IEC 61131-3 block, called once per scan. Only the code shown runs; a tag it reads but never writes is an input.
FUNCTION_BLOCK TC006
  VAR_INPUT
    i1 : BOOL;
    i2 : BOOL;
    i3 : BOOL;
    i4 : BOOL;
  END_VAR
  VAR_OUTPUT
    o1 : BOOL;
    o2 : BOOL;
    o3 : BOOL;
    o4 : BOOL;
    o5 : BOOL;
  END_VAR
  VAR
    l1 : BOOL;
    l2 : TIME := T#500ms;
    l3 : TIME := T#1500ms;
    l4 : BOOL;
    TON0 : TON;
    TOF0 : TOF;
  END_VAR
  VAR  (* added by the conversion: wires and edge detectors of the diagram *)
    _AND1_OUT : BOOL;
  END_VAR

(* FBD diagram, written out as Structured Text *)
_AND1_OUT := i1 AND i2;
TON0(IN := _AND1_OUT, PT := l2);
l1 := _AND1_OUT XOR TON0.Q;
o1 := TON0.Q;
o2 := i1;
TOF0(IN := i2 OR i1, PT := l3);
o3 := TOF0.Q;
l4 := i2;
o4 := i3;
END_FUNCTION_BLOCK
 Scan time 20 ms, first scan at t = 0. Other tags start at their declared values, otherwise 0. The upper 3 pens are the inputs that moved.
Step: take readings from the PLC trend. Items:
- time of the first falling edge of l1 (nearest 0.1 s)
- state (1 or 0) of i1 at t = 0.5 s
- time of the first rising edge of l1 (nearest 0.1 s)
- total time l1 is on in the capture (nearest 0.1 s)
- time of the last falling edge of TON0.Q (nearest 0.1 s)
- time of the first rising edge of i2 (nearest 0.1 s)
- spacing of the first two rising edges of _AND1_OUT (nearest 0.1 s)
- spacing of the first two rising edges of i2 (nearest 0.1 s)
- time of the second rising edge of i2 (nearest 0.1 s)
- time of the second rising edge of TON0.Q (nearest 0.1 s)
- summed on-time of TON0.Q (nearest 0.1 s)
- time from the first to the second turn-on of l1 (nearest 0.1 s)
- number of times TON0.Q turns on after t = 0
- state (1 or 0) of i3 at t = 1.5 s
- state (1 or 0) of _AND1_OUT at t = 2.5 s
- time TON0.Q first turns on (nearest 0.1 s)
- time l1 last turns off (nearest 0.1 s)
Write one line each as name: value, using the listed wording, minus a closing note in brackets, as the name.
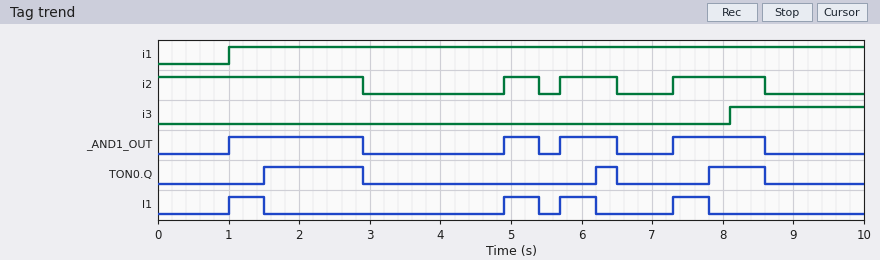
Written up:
time of the first falling edge of l1: 1.5 s
state (1 or 0) of i1 at t = 0.5 s: 0
time of the first rising edge of l1: 1.0 s
total time l1 is on in the capture: 2.0 s
time of the last falling edge of TON0.Q: 8.6 s
time of the first rising edge of i2: 4.9 s
spacing of the first two rising edges of _AND1_OUT: 3.9 s
spacing of the first two rising edges of i2: 0.8 s
time of the second rising edge of i2: 5.7 s
time of the second rising edge of TON0.Q: 6.2 s
summed on-time of TON0.Q: 2.5 s
time from the first to the second turn-on of l1: 3.9 s
number of times TON0.Q turns on after t = 0: 3
state (1 or 0) of i3 at t = 1.5 s: 0
state (1 or 0) of _AND1_OUT at t = 2.5 s: 1
time TON0.Q first turns on: 1.5 s
time l1 last turns off: 7.8 s
